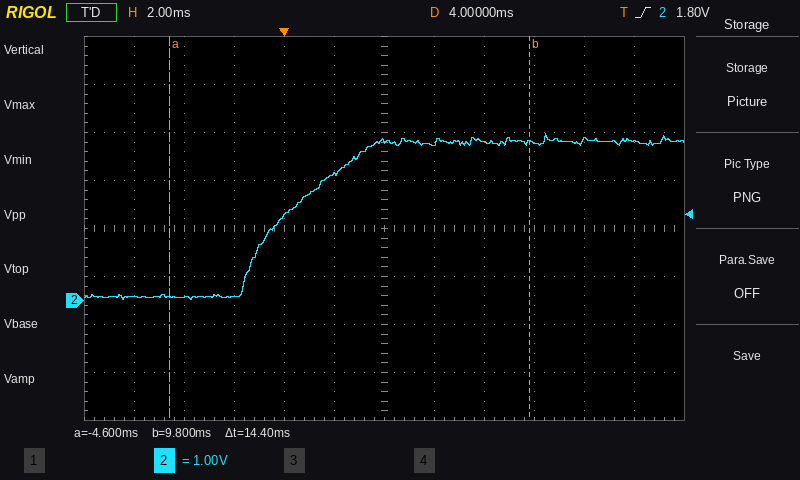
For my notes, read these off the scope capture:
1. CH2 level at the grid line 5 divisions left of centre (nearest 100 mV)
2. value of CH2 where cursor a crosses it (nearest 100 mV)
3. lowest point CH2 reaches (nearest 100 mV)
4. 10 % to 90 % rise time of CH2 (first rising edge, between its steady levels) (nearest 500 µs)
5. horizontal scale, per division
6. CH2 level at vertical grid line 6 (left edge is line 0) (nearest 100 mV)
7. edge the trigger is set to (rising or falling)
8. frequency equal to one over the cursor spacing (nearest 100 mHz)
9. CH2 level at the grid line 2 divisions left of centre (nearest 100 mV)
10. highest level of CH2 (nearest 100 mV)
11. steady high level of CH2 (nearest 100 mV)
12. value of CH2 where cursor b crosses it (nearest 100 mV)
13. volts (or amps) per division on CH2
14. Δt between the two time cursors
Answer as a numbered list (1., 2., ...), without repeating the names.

1. 100 mV
2. 100 mV
3. 0.0 V
4. 4.5 ms
5. 2 ms
6. 3.3 V
7. rising
8. 69.4 Hz
9. 1.8 V
10. 3.5 V
11. 3.3 V
12. 3.3 V
13. 1 V
14. 14.4 ms
